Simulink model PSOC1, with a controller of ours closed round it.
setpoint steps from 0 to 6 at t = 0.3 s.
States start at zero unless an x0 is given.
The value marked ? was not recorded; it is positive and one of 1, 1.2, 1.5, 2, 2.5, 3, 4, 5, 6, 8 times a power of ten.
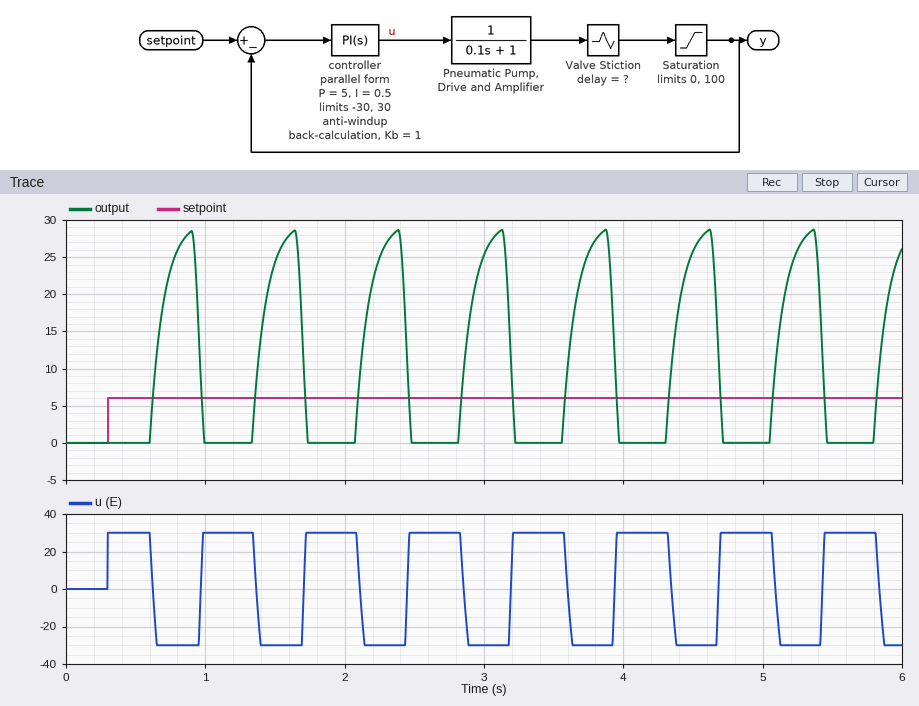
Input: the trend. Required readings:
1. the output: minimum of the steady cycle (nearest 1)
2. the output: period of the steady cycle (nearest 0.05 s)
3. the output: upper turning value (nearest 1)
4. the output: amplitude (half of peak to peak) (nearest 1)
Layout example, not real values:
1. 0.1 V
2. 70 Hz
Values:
1. 0
2. 0.75 s
3. 29
4. 14
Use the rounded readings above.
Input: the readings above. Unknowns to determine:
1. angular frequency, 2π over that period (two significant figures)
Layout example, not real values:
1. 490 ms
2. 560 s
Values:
1. 8.4 rad/s
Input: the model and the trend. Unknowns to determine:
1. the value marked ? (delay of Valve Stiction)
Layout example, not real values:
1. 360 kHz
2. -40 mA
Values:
1. 0.3
